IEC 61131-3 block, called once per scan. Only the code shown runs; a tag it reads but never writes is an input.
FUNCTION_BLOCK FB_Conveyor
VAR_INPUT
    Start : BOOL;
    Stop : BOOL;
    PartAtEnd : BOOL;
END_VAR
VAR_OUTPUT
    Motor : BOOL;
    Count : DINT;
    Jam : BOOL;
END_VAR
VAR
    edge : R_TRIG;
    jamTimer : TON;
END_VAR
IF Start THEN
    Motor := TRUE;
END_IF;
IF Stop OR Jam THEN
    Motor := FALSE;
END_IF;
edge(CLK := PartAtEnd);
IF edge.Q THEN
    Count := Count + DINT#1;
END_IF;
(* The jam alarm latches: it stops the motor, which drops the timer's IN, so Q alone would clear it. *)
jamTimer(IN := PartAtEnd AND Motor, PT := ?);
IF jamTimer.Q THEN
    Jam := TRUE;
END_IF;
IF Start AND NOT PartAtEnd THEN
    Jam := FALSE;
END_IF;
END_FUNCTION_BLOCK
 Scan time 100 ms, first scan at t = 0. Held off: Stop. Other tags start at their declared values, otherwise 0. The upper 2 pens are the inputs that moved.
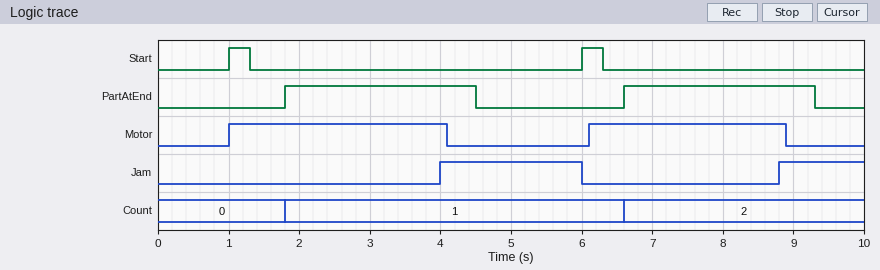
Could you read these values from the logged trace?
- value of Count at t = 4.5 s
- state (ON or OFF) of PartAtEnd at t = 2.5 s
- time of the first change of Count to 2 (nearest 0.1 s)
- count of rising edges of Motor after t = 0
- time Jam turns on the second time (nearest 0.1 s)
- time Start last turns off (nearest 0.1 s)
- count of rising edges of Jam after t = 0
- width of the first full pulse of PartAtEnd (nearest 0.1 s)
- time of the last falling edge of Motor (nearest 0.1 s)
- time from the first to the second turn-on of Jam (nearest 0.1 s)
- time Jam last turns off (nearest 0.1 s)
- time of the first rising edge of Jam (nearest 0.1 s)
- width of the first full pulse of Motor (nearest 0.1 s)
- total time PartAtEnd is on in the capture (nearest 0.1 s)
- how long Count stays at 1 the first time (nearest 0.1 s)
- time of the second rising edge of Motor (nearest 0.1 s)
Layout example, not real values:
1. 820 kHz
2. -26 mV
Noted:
1. 1
2. ON
3. 6.6 s
4. 2
5. 8.8 s
6. 6.3 s
7. 2
8. 2.7 s
9. 8.9 s
10. 4.8 s
11. 6.0 s
12. 4.0 s
13. 3.1 s
14. 5.4 s
15. 4.8 s
16. 6.1 s
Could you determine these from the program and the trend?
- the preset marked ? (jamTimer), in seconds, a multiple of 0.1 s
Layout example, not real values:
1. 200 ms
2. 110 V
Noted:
1. 2.2 s
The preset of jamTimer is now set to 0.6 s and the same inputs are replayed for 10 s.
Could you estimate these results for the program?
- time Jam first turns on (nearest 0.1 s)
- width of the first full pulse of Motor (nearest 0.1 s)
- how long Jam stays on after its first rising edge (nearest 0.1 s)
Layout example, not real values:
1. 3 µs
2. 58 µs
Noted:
1. 2.4 s
2. 1.5 s
3. 3.6 s
